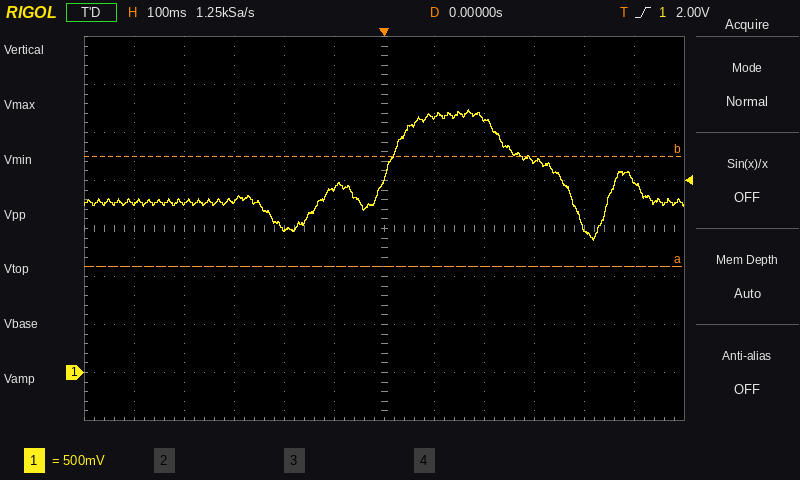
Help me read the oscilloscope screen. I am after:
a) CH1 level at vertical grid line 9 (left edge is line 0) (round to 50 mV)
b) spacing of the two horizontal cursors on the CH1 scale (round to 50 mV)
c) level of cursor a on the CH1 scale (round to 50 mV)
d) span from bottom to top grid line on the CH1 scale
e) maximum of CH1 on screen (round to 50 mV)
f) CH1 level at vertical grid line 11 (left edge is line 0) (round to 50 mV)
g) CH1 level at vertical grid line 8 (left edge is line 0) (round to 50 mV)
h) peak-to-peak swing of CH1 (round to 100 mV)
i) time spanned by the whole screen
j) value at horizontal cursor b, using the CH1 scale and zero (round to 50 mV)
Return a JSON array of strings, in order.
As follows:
["2.20 V", "1.15 V", "1.10 V", "4 V", "2.75 V", "2.00 V", "2.65 V", "1.40 V", "1.2 s", "2.25 V"]
